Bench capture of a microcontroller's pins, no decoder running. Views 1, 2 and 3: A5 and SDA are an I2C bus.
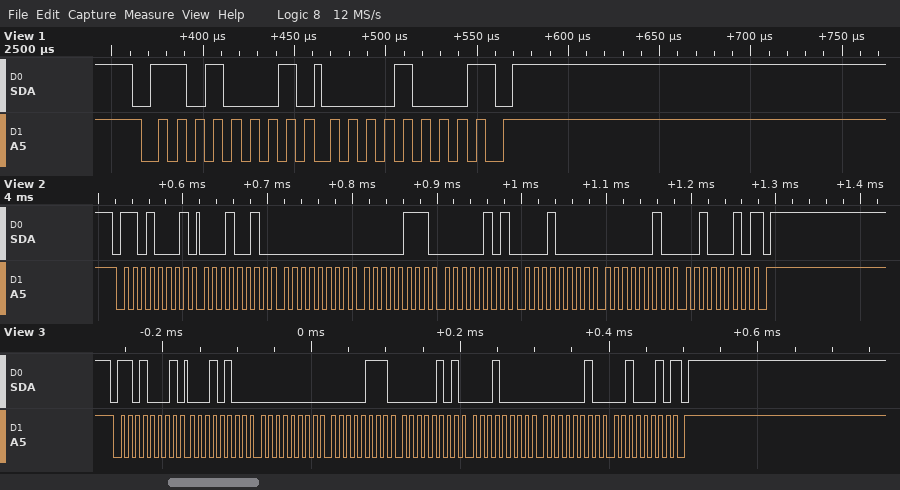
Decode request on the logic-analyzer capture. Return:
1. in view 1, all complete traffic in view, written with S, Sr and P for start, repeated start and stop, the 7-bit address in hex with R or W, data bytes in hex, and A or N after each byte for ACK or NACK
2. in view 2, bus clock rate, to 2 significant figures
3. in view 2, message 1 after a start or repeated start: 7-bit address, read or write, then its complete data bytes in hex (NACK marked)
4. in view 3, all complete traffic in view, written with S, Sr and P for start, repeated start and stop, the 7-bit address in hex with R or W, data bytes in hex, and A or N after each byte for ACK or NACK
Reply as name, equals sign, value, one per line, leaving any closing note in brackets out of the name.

in view 1, all complete traffic in view, written with S, Sr and P for start, repeated start and stop, the 7-bit address in hex with R or W, data bytes in hex, and A or N after each byte for ACK or NACK = S 68R A 08 N P
in view 2, bus clock rate, to 2 significant figures = 100 kHz
in view 2, message 1 after a start or repeated start: 7-bit address, read or write, then its complete data bytes in hex = 0x68 read: 12 00 07 05 10 02 22 NACK
in view 3, all complete traffic in view, written with S, Sr and P for start, repeated start and stop, the 7-bit address in hex with R or W, data bytes in hex, and A or N after each byte for ACK or NACK = S 68R A 14 A 00 A 07 A 05 A 10 A 02 A 22 N P
